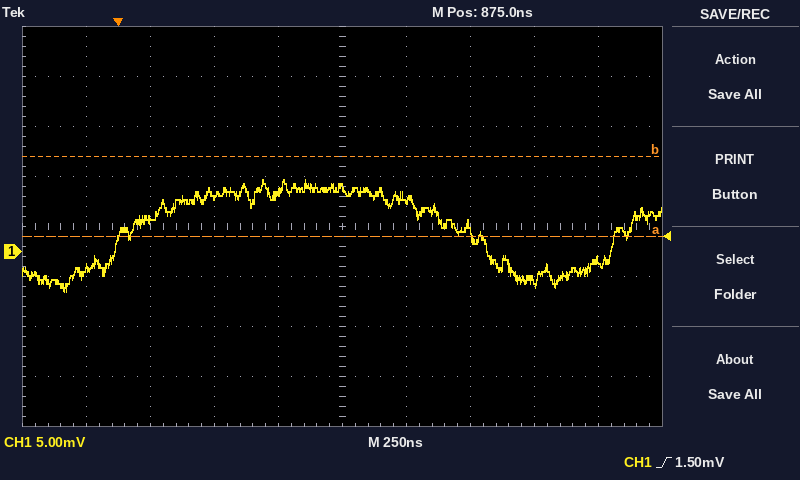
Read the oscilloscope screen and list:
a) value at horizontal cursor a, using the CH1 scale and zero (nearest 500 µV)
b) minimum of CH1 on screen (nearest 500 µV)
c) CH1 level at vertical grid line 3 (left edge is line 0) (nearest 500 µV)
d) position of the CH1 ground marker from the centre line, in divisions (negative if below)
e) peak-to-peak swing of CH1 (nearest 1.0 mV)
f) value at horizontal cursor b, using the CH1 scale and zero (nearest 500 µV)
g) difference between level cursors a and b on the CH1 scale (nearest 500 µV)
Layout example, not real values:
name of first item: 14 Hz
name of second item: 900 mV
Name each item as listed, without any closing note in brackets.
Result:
value at horizontal cursor a, using the CH1 scale and zero: 1.5 mV
minimum of CH1 on screen: -4.0 mV
CH1 level at vertical grid line 3 (left edge is line 0): 5.5 mV
position of the CH1 ground marker from the centre line, in divisions: -0.5 div
peak-to-peak swing of CH1: 11.0 mV
value at horizontal cursor b, using the CH1 scale and zero: 9.5 mV
difference between level cursors a and b on the CH1 scale: 8.0 mV
